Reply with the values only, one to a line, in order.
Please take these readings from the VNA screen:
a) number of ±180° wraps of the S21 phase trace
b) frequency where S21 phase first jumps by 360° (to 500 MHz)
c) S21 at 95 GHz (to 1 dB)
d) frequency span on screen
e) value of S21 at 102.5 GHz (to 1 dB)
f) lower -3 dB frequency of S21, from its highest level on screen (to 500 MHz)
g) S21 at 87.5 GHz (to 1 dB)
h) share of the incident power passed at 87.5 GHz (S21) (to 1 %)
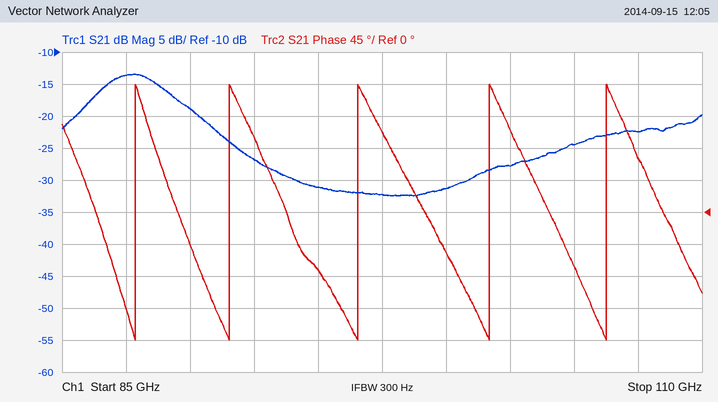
5
88.0 GHz
-31 dB
25 GHz
-28 dB
86.5 GHz
-14 dB
4 %
